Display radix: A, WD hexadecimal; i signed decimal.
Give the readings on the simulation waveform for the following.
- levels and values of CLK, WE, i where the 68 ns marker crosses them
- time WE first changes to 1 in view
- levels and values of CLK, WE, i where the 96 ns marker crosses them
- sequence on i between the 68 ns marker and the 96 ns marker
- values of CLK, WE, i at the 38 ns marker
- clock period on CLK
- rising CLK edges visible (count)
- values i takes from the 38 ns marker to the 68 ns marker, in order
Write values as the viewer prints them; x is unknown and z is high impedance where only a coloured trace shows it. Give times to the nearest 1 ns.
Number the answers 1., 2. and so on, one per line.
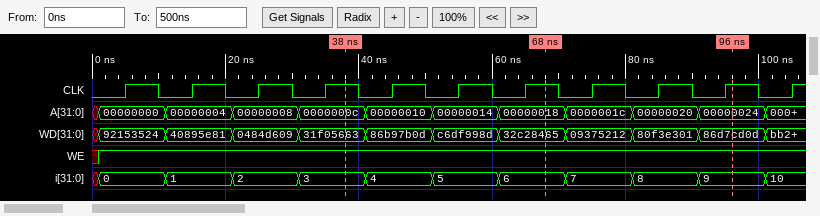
1. CLK=1, WE=1, i=6
2. 1 ns
3. CLK=1, WE=1, i=9
4. 6, 7, 8, 9
5. CLK=1, WE=1, i=3
6. 10 ns
7. 11
8. 3, 4, 5, 6
